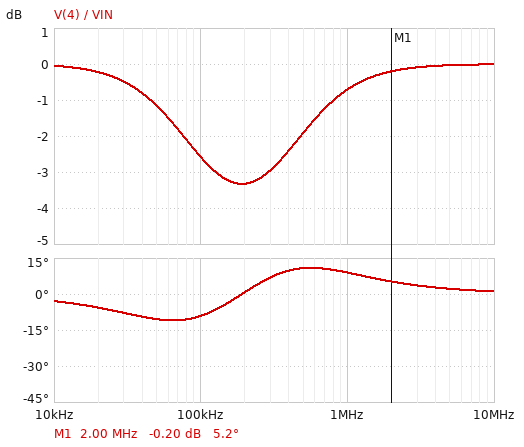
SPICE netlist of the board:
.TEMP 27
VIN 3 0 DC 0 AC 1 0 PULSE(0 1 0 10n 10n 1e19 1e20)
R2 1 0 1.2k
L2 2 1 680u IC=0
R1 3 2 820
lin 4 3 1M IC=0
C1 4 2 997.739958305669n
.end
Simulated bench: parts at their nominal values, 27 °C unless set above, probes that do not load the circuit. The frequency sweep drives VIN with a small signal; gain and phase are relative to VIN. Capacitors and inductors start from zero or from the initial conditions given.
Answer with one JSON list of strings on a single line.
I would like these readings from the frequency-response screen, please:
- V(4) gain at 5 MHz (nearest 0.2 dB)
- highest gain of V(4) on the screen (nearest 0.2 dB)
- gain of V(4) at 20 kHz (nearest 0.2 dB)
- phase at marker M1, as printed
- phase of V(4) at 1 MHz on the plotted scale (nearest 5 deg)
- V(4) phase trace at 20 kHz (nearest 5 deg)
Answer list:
["0 dB", "0 dB", "-0.2 dB", "5.2 deg", "10 deg", "-5 deg"]
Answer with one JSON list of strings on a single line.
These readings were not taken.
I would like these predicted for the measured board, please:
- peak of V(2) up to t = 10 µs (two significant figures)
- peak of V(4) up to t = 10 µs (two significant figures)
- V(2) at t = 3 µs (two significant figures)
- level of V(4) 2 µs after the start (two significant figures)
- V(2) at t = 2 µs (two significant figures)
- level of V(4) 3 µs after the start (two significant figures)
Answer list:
["990 mV", "1.0 V", "890 mV", "830 mV", "830 mV", "890 mV"]
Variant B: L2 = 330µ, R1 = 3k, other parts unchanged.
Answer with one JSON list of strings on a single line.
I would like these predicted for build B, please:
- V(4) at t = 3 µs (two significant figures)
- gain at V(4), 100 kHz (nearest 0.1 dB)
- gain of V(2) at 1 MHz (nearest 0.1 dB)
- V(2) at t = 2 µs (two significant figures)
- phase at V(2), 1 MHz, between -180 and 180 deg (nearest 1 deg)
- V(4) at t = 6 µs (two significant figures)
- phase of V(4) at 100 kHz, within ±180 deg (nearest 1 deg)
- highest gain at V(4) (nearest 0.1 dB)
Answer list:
["930 mV", "-2.1 dB", "-6.2 dB", "850 mV", "18 deg", "990 mV", "-22 deg", "0 dB"]
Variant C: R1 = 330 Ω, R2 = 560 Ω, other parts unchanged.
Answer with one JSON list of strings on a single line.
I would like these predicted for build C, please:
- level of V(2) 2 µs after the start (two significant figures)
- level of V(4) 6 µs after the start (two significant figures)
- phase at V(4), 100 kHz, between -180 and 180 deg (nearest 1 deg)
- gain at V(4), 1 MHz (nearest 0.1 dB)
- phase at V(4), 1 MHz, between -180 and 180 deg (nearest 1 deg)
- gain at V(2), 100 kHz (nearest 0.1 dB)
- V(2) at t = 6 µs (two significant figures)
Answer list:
["760 mV", "880 mV", "3 deg", "-0.1 dB", "4 deg", "-3.0 dB", "870 mV"]
